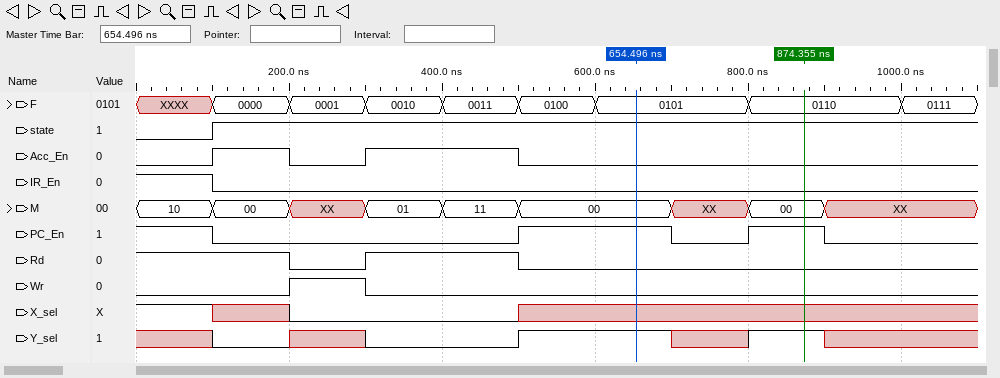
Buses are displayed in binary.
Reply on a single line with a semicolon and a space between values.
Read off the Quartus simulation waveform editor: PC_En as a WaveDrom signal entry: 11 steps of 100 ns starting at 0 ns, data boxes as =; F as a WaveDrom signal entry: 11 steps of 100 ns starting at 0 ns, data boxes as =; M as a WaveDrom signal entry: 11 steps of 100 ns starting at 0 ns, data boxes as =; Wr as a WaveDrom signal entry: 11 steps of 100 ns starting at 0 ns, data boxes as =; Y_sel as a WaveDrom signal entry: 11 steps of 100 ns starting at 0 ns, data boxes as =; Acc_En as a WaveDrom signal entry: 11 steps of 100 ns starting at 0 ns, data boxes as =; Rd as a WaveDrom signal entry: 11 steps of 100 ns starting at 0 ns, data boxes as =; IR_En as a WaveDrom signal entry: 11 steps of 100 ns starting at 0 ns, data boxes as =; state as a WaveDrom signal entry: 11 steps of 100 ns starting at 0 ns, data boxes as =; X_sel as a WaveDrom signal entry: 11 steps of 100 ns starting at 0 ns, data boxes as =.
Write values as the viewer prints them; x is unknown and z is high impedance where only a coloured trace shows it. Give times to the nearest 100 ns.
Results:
{name: 'PC_En', wave: '10...1.010.'}; {name: 'F', wave: 'x======.=.=', data: '0000 0001 0010 0011 0100 0101 0110 0111'}; {name: 'M', wave: '==x===.x=x.', data: '10 00 01 11 00 00'}; {name: 'Wr', wave: '0.10.......'}; {name: 'Y_sel', wave: 'x0x0.1.x1x.'}; {name: 'Acc_En', wave: '0101.0.....'}; {name: 'Rd', wave: '1.01.0.....'}; {name: 'IR_En', wave: '10.........'}; {name: 'state', wave: '01.........'}; {name: 'X_sel', wave: '1x0..x.....'}
